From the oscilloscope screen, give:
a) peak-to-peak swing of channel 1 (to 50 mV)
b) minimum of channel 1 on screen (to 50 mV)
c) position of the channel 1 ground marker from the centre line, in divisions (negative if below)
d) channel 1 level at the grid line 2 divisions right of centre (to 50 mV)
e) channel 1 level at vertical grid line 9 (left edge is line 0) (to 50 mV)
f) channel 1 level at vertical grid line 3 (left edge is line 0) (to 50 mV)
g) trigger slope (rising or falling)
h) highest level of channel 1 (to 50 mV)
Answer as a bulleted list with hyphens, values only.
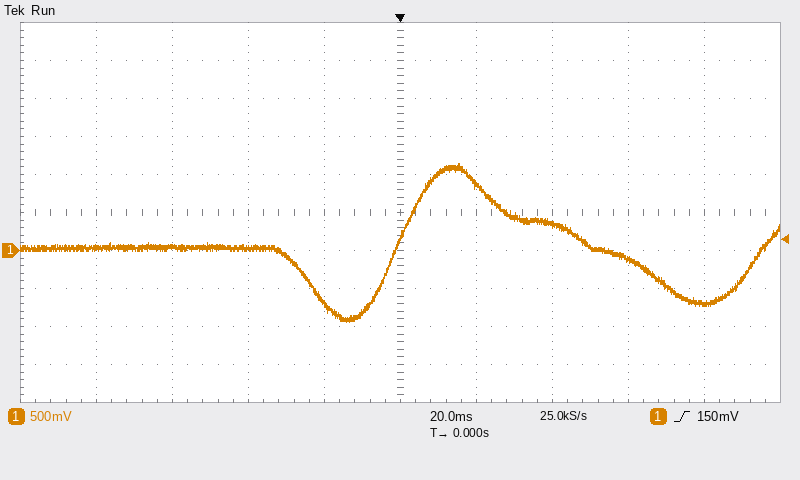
- 2.10 V
- -950 mV
- -1.0 div
- 350 mV
- -700 mV
- 50 mV
- rising
- 1.15 V
